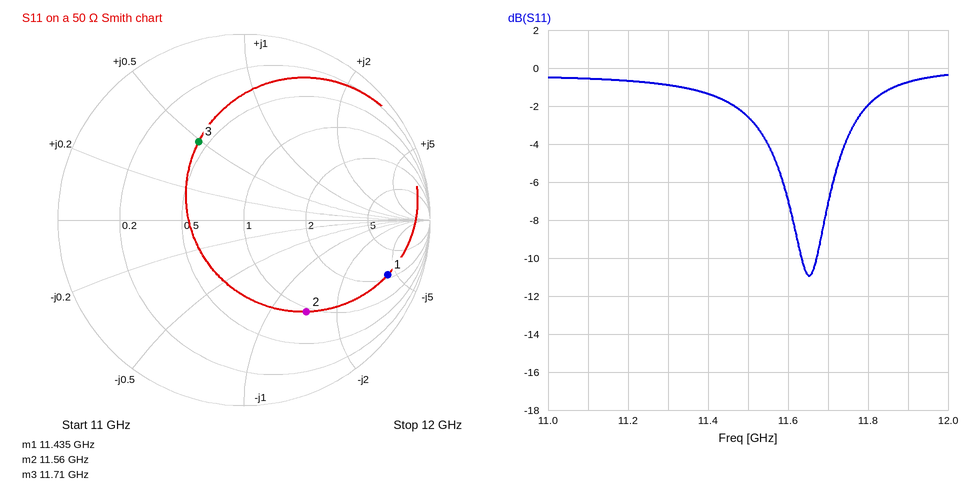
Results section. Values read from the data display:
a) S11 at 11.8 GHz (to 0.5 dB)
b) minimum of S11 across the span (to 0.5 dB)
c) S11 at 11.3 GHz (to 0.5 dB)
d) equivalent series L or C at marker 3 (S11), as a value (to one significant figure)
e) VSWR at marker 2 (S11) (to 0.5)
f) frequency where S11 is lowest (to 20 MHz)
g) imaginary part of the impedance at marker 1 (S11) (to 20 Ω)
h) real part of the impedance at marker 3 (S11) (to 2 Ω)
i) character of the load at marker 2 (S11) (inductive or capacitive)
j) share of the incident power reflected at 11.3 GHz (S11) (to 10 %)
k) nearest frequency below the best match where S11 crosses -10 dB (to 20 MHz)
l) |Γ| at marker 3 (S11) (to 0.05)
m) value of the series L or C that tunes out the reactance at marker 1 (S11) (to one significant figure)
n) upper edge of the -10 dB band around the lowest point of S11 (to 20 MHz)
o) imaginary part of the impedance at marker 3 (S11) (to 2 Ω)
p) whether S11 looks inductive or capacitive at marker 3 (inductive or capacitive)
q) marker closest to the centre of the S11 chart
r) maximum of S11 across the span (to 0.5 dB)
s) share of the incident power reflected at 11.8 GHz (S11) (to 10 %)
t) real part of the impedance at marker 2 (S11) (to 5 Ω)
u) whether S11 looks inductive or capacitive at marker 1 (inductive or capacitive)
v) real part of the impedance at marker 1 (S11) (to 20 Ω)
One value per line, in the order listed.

-2.0 dB
-11.0 dB
-1.0 dB
300 pH
4.0
11.66 GHz
-220 Ω
22 Ω
capacitive
80 %
11.64 GHz
0.50
3 nH
11.68 GHz
+24 Ω
inductive
marker 3
-0.5 dB
60 %
45 Ω
capacitive
120 Ω
